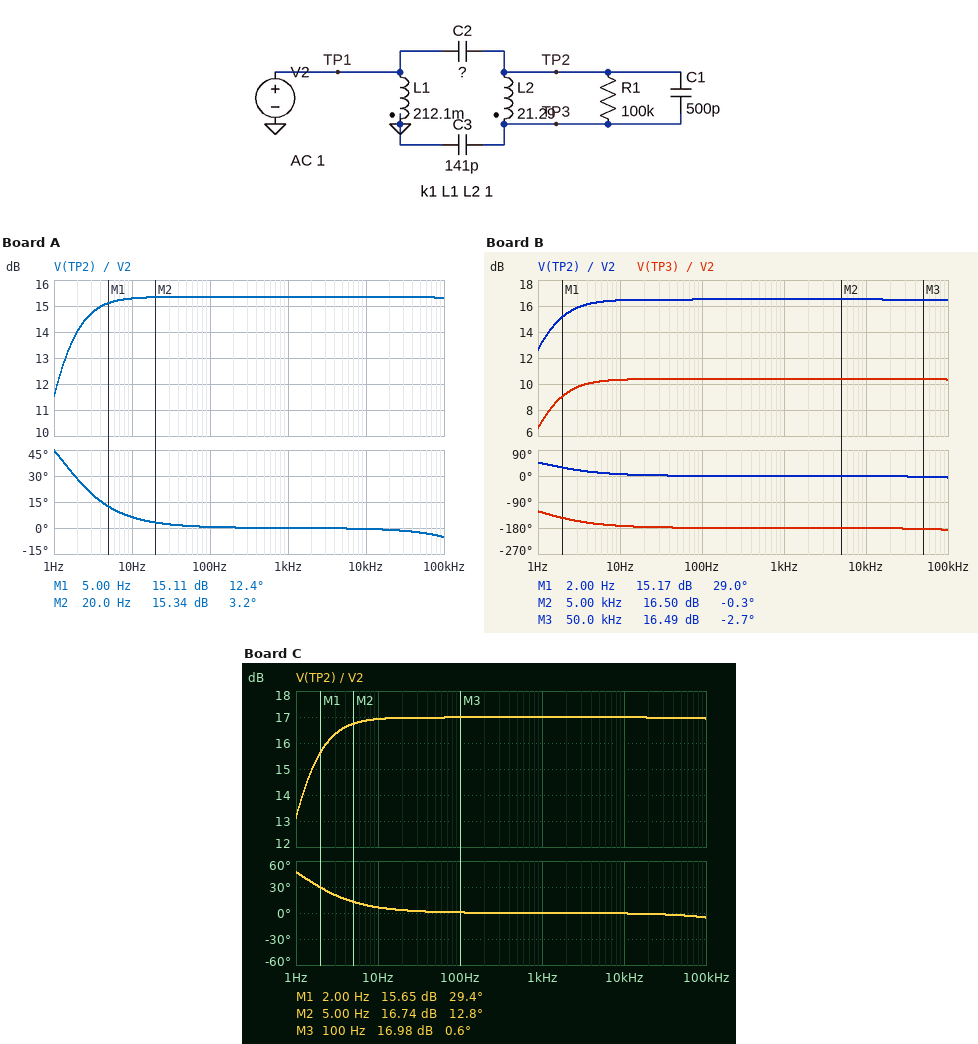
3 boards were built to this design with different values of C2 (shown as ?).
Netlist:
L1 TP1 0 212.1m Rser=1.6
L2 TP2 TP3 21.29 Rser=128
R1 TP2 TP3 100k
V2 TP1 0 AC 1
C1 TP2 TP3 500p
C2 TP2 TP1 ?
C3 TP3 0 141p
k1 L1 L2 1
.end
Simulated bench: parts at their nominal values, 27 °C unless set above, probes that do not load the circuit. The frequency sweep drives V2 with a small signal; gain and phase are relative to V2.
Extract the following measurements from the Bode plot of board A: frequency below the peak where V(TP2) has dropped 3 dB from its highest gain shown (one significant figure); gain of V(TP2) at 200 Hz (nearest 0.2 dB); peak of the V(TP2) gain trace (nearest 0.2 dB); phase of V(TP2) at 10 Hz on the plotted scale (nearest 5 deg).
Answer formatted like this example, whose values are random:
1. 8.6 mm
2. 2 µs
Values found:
1. 1 Hz
2. 15.4 dB
3. 15.4 dB
4. 5 deg
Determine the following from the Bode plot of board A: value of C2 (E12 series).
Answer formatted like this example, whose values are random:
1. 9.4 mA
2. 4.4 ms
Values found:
1. 120 pF
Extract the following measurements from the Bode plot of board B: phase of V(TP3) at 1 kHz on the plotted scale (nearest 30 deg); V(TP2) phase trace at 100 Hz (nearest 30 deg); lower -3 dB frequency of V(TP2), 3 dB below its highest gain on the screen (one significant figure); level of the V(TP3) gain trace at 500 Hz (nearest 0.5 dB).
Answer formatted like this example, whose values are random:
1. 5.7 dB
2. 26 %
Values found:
1. -180 deg
2. 0 deg
3. 1 Hz
4. 10.5 dB
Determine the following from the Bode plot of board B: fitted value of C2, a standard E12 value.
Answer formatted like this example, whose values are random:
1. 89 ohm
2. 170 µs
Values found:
1. 82 pF
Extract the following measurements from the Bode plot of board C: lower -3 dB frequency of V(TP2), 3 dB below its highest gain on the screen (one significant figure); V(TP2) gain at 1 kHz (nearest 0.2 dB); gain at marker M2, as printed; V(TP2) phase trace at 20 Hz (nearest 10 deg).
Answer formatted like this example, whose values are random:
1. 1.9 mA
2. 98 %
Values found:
1. 1 Hz
2. 17.0 dB
3. 16.74 dB
4. 0 deg
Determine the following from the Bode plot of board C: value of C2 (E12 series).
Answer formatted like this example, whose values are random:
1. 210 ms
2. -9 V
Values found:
1. 68 pF
